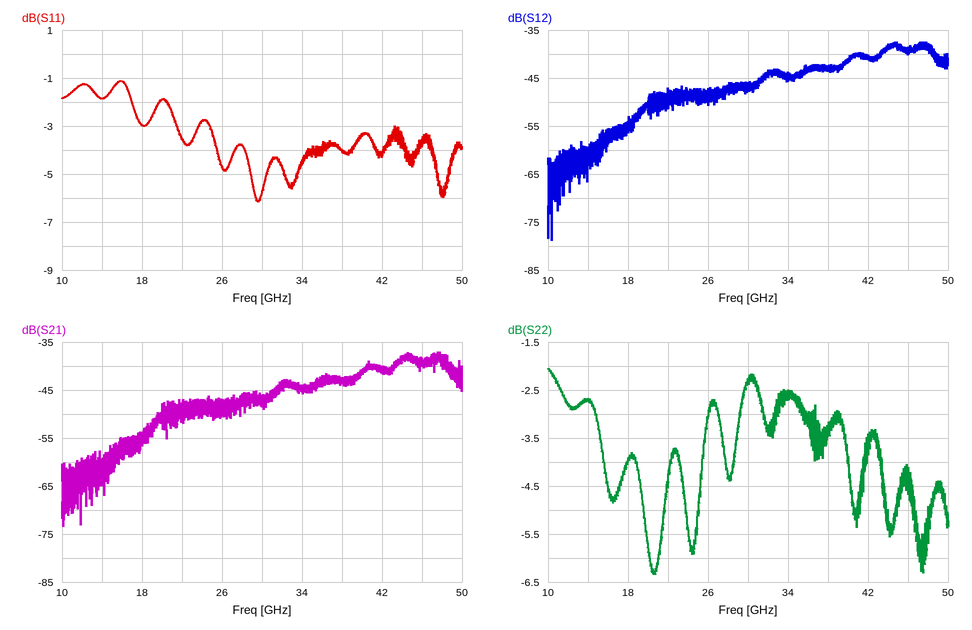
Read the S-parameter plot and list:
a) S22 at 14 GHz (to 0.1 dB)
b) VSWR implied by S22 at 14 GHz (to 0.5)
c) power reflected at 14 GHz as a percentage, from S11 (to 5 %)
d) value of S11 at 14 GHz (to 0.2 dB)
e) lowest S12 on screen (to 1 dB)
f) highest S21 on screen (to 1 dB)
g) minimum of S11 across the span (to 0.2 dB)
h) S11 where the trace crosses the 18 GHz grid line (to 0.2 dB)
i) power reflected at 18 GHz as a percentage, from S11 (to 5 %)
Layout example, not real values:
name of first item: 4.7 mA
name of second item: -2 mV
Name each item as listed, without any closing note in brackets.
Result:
S22 at 14 GHz: -2.7 dB
VSWR implied by S22 at 14 GHz: 6.5
power reflected at 14 GHz as a percentage, from S11: 65 %
value of S11 at 14 GHz: -1.8 dB
lowest S12 on screen: -79 dB
highest S21 on screen: -37 dB
minimum of S11 across the span: -6.2 dB
S11 where the trace crosses the 18 GHz grid line: -3.0 dB
power reflected at 18 GHz as a percentage, from S11: 50 %
